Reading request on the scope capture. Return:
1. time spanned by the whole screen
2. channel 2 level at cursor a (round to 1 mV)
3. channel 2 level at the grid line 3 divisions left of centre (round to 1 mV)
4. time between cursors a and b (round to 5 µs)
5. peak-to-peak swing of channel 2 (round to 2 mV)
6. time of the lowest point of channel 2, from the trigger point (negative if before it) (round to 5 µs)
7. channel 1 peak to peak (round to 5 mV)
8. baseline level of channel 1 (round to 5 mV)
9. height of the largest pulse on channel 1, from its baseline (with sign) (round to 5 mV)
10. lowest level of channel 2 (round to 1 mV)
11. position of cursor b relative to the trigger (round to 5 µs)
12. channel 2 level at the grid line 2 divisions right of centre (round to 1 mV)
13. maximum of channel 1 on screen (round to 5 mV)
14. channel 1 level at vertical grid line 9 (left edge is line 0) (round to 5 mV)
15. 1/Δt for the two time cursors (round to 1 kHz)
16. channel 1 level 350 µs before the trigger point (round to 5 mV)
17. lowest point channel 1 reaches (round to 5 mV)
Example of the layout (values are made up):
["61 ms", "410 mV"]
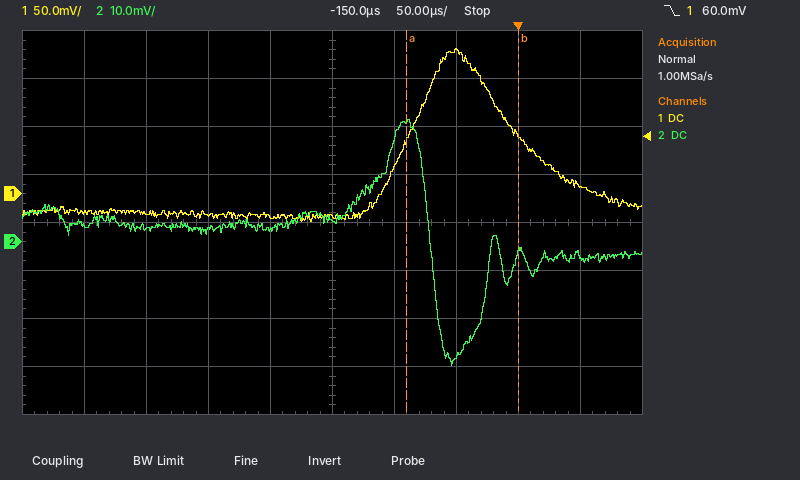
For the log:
["500 µs", "25 mV", "3 mV", "90 µs", "52 mV", "-55 µs", "180 mV", "-20 mV", "+170 mV", "-26 mV", "0 µs", "-24 mV", "150 mV", "10 mV", "11 kHz", "-20 mV", "-30 mV"]
